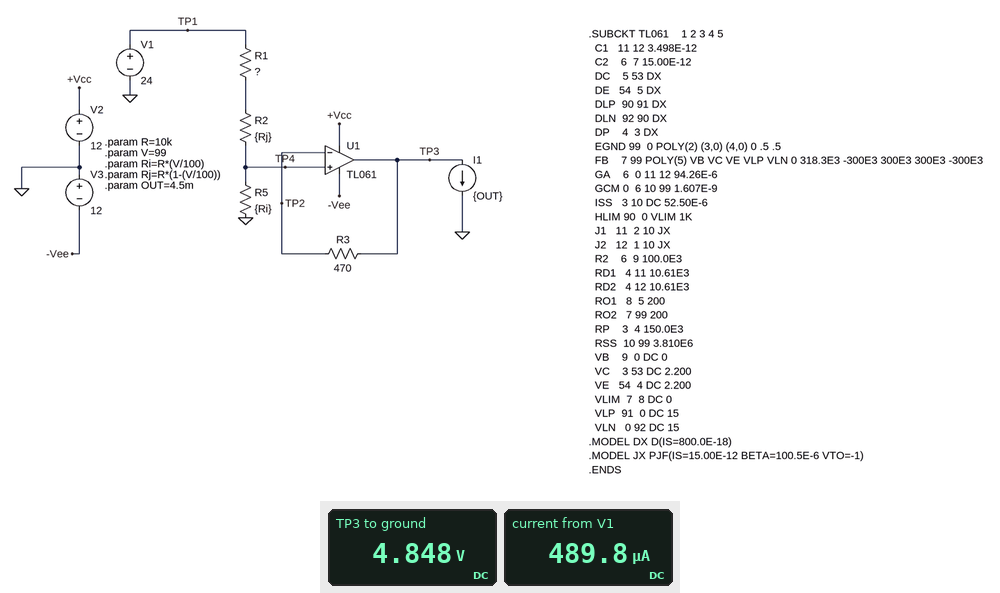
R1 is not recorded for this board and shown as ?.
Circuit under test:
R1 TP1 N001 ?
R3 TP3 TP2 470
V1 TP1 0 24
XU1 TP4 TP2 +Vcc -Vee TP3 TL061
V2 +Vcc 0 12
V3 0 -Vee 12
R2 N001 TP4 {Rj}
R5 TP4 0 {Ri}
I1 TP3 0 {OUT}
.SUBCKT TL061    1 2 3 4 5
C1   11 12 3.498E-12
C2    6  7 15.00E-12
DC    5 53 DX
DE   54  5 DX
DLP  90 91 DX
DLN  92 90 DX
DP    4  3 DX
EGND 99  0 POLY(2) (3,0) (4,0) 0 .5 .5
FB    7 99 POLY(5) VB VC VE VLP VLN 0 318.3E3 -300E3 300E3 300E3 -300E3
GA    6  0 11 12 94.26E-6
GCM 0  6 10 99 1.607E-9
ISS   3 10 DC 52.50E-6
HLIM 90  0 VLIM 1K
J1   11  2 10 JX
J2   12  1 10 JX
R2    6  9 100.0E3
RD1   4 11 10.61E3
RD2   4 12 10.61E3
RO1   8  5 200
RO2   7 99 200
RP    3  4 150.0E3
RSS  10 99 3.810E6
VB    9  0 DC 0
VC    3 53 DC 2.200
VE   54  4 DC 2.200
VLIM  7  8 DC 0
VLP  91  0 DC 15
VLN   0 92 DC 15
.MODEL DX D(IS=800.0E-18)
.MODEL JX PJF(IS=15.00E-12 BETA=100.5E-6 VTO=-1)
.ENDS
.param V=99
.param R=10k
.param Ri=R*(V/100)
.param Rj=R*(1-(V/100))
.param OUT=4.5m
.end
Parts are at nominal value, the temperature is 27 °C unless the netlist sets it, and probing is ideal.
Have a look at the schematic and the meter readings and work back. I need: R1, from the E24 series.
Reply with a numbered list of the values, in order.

1. 39 kΩ
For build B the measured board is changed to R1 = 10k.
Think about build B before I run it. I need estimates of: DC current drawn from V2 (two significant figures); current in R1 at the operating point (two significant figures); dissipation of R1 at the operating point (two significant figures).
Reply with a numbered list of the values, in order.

1. 160 µA
2. 1.2 mA
3. 14 mW
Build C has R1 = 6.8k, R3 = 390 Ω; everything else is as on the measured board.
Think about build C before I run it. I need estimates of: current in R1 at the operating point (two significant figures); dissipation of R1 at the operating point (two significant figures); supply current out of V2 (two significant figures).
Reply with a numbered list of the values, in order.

1. 1.4 mA
2. 14 mW
3. 160 µA
